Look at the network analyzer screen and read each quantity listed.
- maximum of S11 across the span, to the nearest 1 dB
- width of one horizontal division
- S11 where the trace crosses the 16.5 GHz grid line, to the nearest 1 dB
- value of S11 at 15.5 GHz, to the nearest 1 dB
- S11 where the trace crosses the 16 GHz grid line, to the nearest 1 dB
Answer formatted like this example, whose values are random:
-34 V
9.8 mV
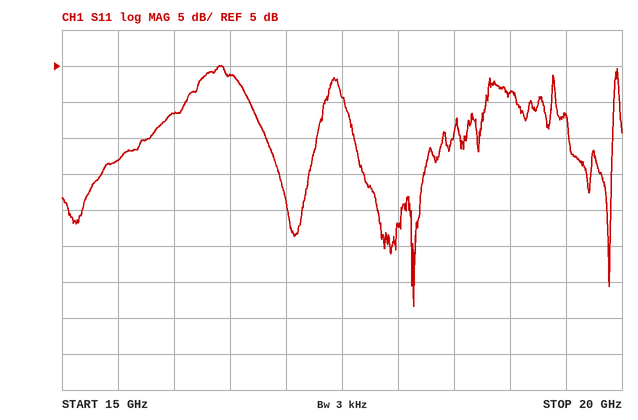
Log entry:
5 dB
500 MHz
4 dB
-8 dB
-2 dB
